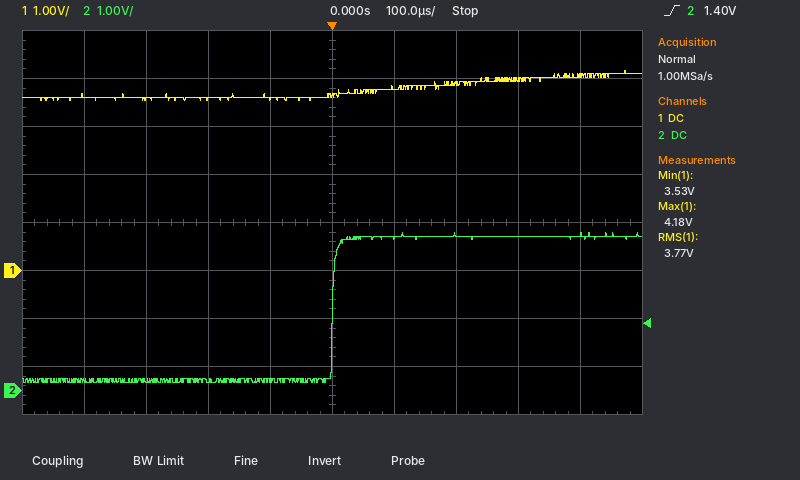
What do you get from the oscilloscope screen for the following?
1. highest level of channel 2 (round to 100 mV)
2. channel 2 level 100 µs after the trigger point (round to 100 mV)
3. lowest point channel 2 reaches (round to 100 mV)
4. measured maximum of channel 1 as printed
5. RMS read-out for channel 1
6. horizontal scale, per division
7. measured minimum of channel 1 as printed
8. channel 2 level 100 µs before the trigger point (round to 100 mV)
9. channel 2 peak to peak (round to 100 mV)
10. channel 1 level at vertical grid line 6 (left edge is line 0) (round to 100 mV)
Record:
3.3 V
3.2 V
200 mV
4.18 V
3.77 V
100 µs
3.53 V
200 mV
3.1 V
3.8 V
